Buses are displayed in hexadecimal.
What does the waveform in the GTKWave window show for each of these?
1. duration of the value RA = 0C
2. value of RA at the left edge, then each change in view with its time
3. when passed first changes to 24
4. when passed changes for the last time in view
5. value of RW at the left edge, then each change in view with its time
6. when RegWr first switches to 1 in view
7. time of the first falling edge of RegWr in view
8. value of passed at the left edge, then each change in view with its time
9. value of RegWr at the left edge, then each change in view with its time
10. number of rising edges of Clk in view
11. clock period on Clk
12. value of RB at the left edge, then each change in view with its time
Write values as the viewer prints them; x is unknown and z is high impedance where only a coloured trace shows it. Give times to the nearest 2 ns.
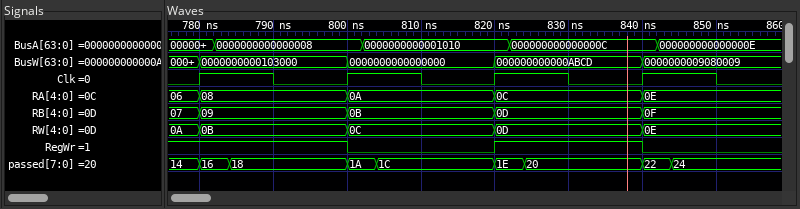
20 ns
06, 08 at 780 ns, 0A at 800 ns, 0C at 820 ns, 0E at 840 ns
844 ns
844 ns
0A, 0B at 780 ns, 0C at 800 ns, 0D at 820 ns, 0E at 840 ns
820 ns
800 ns
14, 16 at 780 ns, 18 at 784 ns, 1A at 800 ns, 1C at 804 ns, 1E at 820 ns, 20 at 824 ns, 22 at 840 ns, 24 at 844 ns
1, 0 at 800 ns, 1 at 820 ns, 0 at 840 ns
4
20 ns
07, 09 at 780 ns, 0B at 800 ns, 0D at 820 ns, 0F at 840 ns
